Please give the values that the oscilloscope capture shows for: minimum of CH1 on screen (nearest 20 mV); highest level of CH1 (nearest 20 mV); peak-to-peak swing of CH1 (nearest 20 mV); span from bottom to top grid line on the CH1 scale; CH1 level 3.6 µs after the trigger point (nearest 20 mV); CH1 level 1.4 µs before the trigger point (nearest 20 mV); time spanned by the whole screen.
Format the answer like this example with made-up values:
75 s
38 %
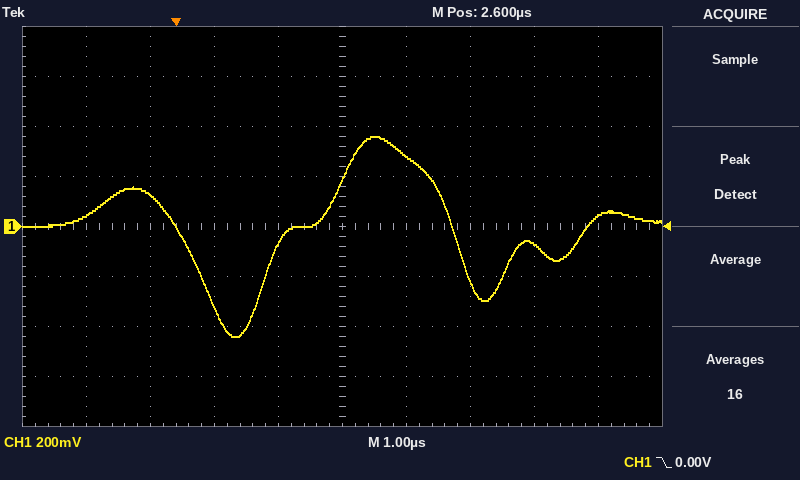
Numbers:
-440 mV
360 mV
800 mV
1.6 V
280 mV
40 mV
10 µs
